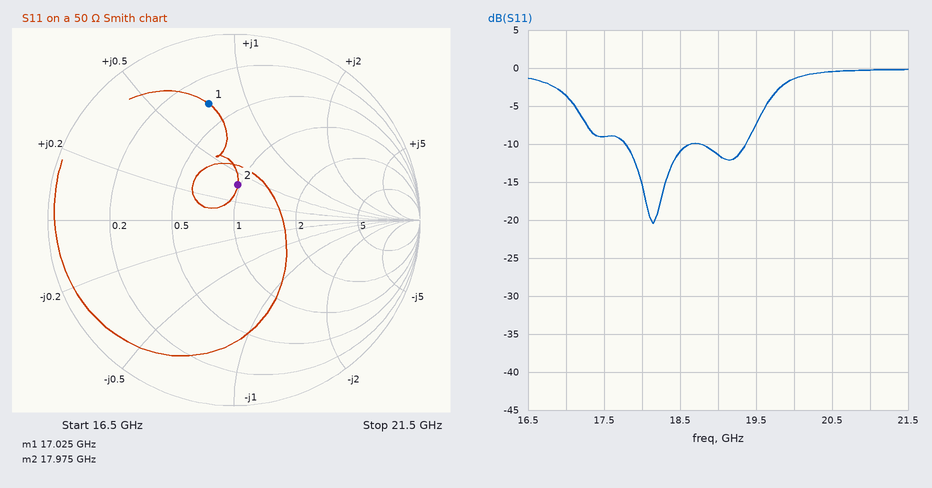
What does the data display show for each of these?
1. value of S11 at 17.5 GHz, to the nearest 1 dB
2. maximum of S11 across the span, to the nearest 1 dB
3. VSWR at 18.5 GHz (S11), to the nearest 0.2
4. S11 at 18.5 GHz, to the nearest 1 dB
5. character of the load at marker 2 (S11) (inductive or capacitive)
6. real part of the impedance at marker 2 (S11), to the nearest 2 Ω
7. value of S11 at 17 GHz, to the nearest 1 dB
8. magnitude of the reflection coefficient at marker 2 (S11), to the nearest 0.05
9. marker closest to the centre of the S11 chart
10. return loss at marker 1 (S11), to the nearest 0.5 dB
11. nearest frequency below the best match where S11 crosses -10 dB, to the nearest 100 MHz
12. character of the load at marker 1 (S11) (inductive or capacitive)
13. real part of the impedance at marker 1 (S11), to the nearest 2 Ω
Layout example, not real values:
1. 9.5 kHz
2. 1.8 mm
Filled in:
1. -9 dB
2. 0 dB
3. 1.8
4. -11 dB
5. inductive
6. 48 Ω
7. -4 dB
8. 0.20
9. marker 2
10. 4.0 dB
11. 17.8 GHz
12. inductive
13. 18 Ω
